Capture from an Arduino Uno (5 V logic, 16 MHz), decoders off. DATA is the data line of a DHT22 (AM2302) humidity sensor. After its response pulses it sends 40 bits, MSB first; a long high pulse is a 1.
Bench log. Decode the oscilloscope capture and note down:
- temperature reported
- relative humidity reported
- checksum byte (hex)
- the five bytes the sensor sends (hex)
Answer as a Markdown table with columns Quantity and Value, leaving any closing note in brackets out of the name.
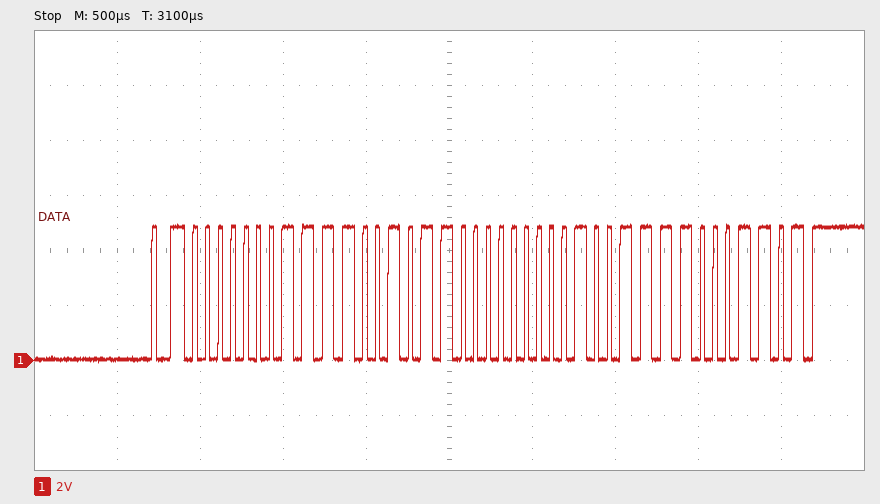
| Quantity | Value |
|---|---|
| temperature reported | -3.9 °C |
| relative humidity reported | 48.5 % |
| checksum byte | 0x8D |
| the five bytes the sensor sends | 01 E5 80 27 8D |
